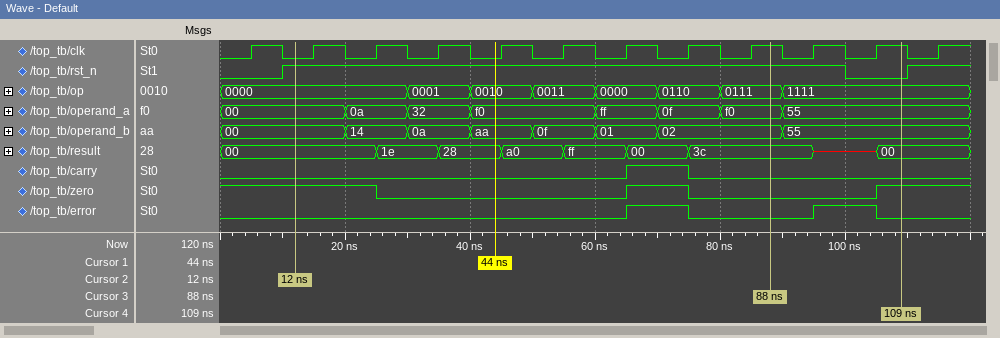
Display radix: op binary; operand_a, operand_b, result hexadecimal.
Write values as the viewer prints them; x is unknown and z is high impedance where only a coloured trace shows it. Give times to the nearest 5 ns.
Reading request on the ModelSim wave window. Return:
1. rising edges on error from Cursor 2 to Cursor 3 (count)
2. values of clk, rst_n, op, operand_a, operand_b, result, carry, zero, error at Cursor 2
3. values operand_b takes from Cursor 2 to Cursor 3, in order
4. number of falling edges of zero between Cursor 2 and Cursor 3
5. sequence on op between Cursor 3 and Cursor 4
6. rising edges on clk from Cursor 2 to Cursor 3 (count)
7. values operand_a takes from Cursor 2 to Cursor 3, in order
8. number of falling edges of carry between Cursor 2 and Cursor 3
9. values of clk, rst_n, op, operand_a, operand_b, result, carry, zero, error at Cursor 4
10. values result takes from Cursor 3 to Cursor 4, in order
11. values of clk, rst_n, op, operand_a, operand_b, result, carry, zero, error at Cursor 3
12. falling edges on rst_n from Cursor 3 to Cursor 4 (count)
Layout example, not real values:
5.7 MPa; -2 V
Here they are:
1; clk=0, rst_n=1, op=0000, operand_a=00, operand_b=00, result=00, carry=0, zero=1, error=0; 00, 14, 0a, aa, 0f, 01, 02; 2; 0111, 1111; 8; 00, 0a, 32, f0, ff, 0f, f0; 1; clk=1, rst_n=0, op=1111, operand_a=55, operand_b=55, result=00, carry=0, zero=1, error=0; 3c, x, 00; clk=1, rst_n=1, op=0111, operand_a=f0, operand_b=02, result=3c, carry=0, zero=0, error=0; 1
